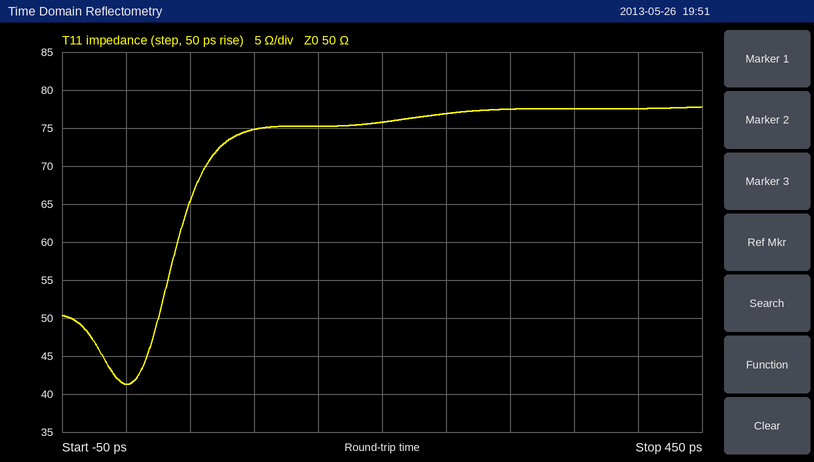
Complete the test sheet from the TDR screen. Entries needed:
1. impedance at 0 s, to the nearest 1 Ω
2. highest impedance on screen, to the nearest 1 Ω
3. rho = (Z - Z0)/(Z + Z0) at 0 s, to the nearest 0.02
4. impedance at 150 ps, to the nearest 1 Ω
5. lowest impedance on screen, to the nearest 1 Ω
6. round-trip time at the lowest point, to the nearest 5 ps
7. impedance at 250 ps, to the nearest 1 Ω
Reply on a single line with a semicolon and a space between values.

41 Ω; 78 Ω; -0.10; 75 Ω; 41 Ω; 0 ps; 77 Ω
